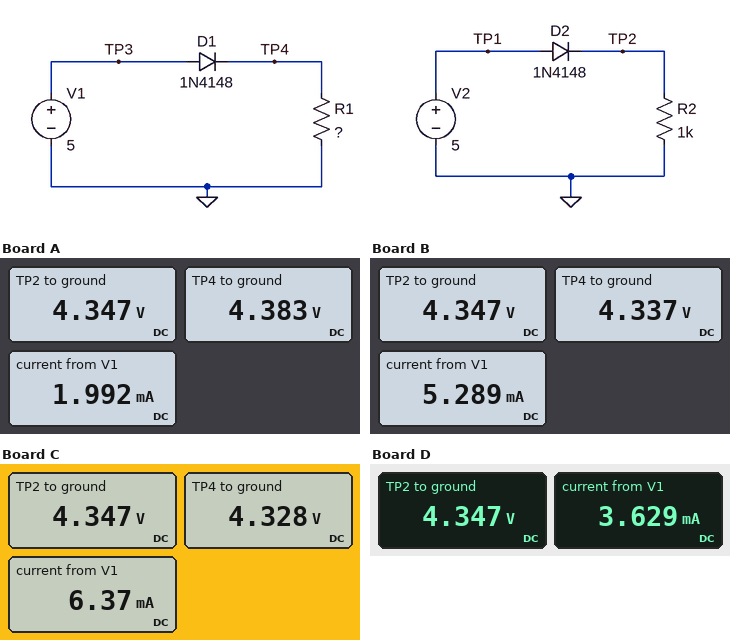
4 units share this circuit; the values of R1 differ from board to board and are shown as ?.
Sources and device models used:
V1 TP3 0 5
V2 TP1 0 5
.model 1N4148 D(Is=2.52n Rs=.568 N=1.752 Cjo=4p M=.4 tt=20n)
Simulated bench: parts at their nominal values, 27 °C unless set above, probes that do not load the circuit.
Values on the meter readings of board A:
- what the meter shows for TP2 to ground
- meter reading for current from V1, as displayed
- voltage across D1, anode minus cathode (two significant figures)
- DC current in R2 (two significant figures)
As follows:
4.347 V
1.992 mA
620 mV
4.3 mA
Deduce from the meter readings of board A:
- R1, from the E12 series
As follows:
2.2 kΩ
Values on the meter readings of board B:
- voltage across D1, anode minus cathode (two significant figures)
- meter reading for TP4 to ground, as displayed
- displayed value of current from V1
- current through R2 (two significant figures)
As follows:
660 mV
4.337 V
5.289 mA
4.3 mA
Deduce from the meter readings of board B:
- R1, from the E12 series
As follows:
820 Ω
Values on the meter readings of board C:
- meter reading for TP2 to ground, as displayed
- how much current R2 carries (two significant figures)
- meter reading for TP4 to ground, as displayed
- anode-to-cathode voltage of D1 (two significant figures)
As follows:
4.347 V
4.3 mA
4.328 V
670 mV
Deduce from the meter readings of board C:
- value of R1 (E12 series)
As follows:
680 Ω
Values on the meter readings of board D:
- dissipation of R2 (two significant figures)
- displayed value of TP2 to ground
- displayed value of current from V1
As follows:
19 mW
4.347 V
3.629 mA
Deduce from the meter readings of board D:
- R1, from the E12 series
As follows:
1.2 kΩ
